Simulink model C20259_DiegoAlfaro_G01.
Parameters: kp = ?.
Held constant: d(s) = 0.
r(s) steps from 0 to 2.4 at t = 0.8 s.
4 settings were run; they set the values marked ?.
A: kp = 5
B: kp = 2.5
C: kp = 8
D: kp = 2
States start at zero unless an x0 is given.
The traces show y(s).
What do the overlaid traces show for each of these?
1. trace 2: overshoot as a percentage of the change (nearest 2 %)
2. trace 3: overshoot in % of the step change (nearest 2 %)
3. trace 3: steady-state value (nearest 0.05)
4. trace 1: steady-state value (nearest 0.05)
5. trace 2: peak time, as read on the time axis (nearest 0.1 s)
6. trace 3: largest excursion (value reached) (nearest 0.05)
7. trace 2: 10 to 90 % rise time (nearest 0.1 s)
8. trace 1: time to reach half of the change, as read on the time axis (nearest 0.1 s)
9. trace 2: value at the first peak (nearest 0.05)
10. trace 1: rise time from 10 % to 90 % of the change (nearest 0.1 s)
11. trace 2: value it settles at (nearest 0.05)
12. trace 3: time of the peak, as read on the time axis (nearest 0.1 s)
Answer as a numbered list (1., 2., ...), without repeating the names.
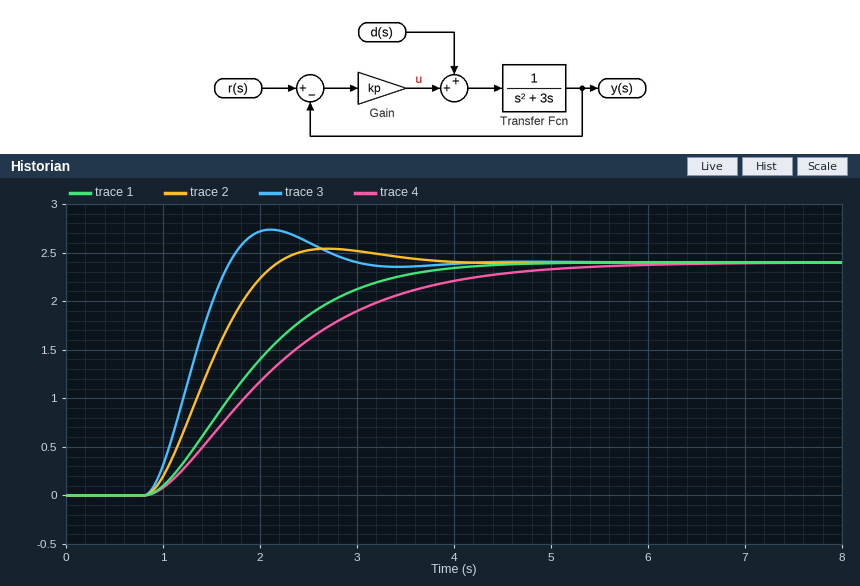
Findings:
1. 6 %
2. 14 %
3. 2.40
4. 2.40
5. 2.7 s
6. 2.75
7. 0.9 s
8. 1.8 s
9. 2.55
10. 2.0 s
11. 2.40
12. 2.1 s
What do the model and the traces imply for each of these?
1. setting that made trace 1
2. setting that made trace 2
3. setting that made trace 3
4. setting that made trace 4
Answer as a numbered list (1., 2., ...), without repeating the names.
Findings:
1. B
2. A
3. C
4. D
